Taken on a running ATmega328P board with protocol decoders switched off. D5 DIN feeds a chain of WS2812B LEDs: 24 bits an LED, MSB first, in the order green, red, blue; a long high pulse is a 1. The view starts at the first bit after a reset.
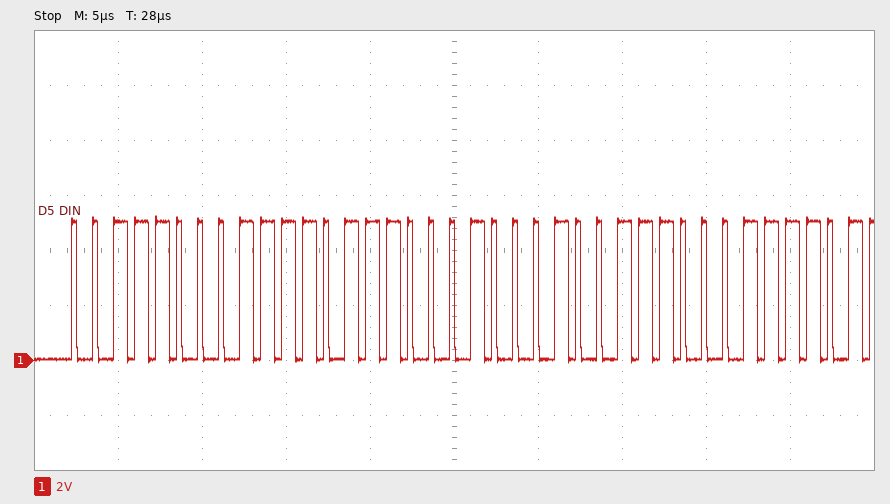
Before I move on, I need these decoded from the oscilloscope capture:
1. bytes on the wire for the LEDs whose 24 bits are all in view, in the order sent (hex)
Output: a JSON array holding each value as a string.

["38 F7 11"]
